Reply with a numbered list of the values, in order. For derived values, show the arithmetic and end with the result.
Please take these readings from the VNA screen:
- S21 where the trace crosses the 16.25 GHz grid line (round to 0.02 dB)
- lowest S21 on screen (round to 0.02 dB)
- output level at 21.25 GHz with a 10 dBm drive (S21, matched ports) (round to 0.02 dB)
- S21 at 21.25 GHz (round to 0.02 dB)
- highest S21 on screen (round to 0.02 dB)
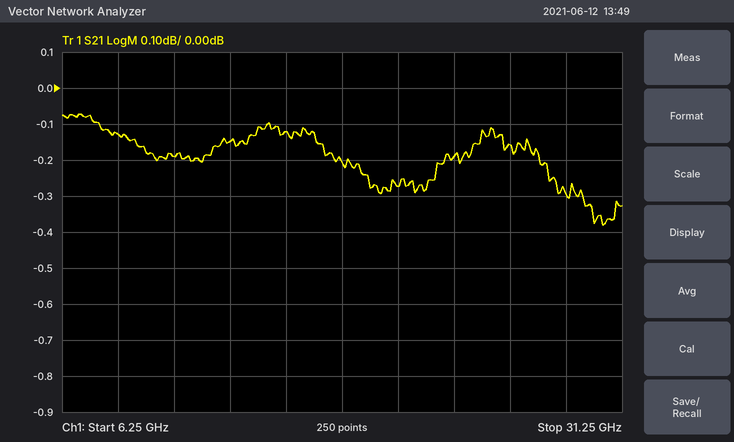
1. -0.12 dB
2. -0.38 dB
3. 10 dBm + (-0.28 dB) = 9.72 dBm
4. -0.28 dB
5. -0.08 dB
